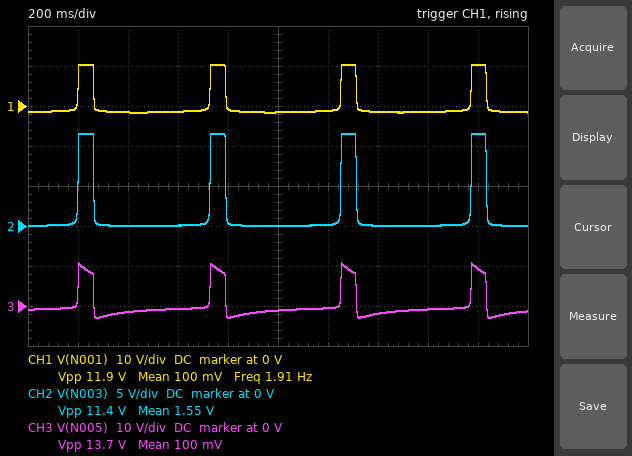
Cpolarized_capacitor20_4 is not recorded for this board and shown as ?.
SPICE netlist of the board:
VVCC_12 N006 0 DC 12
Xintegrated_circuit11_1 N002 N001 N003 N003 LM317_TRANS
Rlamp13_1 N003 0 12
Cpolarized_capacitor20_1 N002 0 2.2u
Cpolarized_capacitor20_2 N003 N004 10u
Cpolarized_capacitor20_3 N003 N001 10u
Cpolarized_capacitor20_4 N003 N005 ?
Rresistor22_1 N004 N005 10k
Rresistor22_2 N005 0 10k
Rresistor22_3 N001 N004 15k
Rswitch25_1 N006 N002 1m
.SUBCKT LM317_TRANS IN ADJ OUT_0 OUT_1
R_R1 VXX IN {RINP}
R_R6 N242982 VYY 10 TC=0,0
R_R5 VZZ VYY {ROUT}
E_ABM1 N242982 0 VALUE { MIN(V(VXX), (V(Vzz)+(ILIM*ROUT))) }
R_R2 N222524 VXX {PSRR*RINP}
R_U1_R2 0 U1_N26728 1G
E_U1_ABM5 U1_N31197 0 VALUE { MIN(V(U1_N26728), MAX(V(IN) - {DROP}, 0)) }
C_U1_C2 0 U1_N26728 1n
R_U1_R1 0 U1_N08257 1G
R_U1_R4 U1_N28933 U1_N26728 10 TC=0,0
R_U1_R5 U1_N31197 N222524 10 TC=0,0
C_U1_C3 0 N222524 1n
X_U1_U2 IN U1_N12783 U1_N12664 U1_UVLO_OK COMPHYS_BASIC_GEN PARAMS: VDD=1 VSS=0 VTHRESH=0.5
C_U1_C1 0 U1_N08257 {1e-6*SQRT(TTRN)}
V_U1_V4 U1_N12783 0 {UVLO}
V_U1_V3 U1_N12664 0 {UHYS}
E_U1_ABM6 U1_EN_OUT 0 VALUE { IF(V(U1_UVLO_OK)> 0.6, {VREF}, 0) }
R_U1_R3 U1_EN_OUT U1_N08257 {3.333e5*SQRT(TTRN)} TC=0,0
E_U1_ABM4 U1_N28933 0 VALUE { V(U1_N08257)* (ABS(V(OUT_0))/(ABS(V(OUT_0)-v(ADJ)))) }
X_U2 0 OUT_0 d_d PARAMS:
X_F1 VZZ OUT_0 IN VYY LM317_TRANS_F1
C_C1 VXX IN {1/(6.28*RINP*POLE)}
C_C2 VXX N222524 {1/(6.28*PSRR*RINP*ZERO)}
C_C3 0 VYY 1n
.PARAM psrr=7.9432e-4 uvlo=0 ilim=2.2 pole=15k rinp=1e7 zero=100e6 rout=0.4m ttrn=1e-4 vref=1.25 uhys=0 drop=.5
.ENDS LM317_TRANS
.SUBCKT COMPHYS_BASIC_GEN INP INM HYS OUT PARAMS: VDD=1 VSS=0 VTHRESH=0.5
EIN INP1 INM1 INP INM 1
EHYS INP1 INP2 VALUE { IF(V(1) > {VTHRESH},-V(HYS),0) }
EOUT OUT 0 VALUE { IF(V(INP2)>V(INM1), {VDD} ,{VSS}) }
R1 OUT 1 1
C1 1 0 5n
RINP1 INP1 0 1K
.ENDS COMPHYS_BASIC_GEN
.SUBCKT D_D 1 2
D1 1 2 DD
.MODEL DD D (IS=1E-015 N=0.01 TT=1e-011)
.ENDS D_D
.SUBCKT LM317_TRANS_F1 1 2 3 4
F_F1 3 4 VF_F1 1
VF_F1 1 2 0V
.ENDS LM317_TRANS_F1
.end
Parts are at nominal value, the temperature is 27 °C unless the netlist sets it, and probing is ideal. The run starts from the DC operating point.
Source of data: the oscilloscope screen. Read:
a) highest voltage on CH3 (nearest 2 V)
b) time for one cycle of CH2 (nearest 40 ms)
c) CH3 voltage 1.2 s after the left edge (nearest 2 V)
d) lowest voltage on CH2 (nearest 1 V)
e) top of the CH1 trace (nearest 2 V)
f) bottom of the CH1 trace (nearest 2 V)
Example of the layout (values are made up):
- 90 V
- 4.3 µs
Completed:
- 10 V
- 520 ms
- 0 V
- 0 V
- 10 V
- -2 V
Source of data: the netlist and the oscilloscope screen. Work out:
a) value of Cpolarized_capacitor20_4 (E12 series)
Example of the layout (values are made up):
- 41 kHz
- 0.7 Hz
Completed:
- 18 µF
